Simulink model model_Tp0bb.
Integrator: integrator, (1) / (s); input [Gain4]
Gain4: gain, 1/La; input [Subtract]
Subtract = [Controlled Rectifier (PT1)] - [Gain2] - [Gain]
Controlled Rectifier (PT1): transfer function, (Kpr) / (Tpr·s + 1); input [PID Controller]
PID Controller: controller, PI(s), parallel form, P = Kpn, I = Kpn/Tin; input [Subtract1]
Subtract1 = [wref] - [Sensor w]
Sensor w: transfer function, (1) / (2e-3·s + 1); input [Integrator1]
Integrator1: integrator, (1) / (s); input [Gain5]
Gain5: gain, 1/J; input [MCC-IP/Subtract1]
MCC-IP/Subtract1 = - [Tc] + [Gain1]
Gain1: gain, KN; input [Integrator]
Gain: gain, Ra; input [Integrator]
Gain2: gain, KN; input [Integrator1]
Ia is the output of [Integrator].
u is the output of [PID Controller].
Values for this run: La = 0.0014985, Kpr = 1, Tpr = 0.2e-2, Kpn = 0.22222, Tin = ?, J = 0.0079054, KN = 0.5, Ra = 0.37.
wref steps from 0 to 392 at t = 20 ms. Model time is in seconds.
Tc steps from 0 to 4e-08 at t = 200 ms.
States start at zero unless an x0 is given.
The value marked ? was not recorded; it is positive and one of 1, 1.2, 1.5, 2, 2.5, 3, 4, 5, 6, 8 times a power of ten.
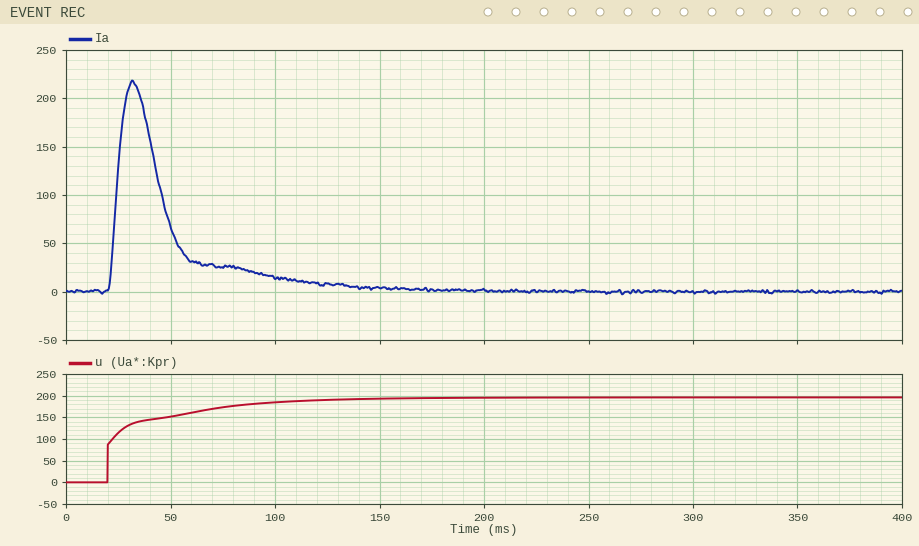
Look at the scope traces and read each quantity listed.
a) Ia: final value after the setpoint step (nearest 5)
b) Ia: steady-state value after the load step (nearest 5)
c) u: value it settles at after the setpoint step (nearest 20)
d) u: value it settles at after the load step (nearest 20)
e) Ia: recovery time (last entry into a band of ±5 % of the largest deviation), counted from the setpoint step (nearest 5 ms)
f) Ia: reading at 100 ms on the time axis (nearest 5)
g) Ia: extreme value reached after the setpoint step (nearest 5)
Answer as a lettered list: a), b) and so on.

a) 0
b) 0
c) 200
d) 200
e) 90 ms
f) 15
g) 215
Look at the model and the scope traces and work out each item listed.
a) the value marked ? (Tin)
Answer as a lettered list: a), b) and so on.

a) 0.015
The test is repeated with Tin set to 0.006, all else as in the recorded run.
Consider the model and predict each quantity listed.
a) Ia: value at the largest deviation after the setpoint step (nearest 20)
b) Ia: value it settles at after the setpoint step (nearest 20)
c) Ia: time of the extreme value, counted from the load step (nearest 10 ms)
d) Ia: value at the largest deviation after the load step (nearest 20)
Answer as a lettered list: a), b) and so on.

a) 360
b) 0
c) 30 ms
d) 0
